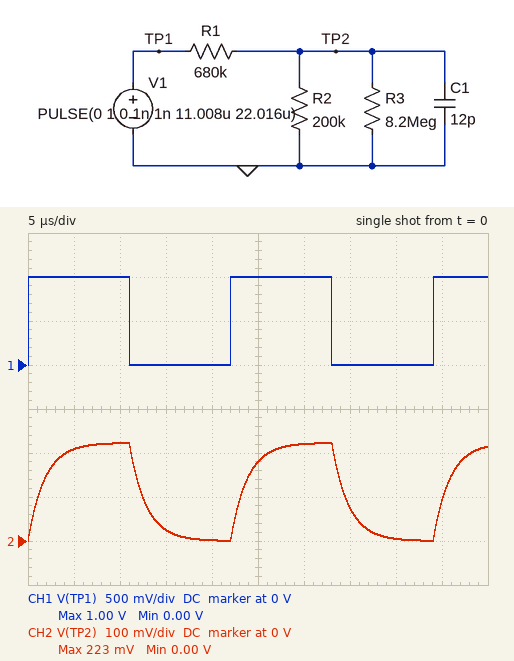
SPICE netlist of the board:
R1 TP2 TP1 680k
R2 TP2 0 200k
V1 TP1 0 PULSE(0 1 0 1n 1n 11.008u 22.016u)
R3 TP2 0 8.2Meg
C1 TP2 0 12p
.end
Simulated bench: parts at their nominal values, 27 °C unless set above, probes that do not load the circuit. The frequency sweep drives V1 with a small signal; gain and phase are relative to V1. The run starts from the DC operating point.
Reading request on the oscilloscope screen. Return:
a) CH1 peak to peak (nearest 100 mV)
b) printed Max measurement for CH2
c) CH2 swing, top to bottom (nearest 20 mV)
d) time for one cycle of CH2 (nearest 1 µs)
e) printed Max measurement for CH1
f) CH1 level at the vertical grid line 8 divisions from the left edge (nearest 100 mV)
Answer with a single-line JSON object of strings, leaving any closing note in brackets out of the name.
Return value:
{"CH1 peak to peak": "1.0 V", "printed Max measurement for CH2": "223 mV", "CH2 swing, top to bottom": "220 mV", "time for one cycle of CH2": "22 µs", "printed Max measurement for CH1": "1.00 V", "CH1 level at the vertical grid line 8 divisions from the left edge": "0 V"}
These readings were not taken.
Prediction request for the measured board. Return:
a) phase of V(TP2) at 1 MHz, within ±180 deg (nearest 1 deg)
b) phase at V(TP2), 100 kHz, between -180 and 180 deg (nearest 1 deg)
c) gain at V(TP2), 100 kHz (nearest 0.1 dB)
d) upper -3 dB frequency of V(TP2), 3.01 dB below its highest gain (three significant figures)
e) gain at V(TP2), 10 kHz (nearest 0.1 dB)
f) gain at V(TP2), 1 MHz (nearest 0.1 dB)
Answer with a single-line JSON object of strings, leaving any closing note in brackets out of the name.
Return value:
{"phase of V(TP2) at 1 MHz, within ±180 deg": "-85 deg", "phase at V(TP2), 100 kHz, between -180 and 180 deg": "-49 deg", "gain at V(TP2), 100 kHz": "-16.7 dB", "upper -3 dB frequency of V(TP2), 3.01 dB below its highest gain": "87.4 kHz", "gain at V(TP2), 10 kHz": "-13.1 dB", "gain at V(TP2), 1 MHz": "-34.2 dB"}
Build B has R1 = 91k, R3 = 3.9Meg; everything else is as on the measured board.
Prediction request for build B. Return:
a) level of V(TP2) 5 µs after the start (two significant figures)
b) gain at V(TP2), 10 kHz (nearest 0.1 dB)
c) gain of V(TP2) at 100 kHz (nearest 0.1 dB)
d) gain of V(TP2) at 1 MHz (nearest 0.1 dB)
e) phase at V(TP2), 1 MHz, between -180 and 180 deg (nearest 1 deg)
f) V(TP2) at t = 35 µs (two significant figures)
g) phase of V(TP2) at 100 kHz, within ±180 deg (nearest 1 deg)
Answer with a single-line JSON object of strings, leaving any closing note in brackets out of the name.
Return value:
{"level of V(TP2) 5 µs after the start": "680 mV", "gain at V(TP2), 10 kHz": "-3.4 dB", "gain of V(TP2) at 100 kHz": "-4.2 dB", "gain of V(TP2) at 1 MHz": "-16.9 dB", "phase at V(TP2), 1 MHz, between -180 and 180 deg": "-78 deg", "V(TP2) at t = 35 µs": "47 mV", "phase of V(TP2) at 100 kHz, within ±180 deg": "-25 deg"}
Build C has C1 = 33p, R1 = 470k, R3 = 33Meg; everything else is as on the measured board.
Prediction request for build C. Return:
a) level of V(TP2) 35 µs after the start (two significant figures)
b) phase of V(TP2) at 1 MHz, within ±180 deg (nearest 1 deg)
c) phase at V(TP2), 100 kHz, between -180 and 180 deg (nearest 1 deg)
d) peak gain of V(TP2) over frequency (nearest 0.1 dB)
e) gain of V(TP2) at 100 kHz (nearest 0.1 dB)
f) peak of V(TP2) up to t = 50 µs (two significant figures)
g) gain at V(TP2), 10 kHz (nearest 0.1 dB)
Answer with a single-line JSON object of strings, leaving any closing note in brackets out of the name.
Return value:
{"level of V(TP2) 35 µs after the start": "180 mV", "phase of V(TP2) at 1 MHz, within ±180 deg": "-88 deg", "phase at V(TP2), 100 kHz, between -180 and 180 deg": "-71 deg", "peak gain of V(TP2) over frequency": "-10.5 dB", "gain of V(TP2) at 100 kHz": "-20.3 dB", "peak of V(TP2) up to t = 50 µs": "270 mV", "gain at V(TP2), 10 kHz": "-10.9 dB"}
